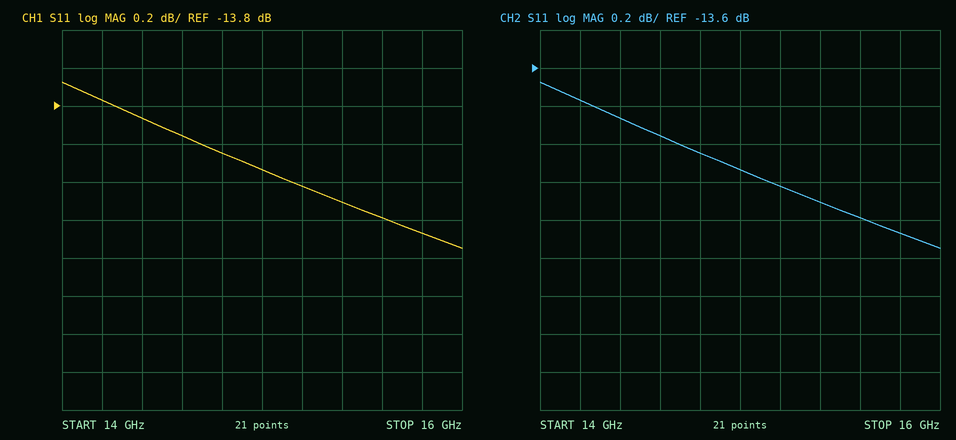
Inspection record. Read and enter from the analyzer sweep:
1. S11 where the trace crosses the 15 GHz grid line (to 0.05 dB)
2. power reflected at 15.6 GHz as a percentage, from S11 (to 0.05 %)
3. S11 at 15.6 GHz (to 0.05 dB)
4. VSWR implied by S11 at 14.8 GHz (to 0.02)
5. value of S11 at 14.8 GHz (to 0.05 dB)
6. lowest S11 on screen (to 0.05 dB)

-14.15 dB
3.65 %
-14.40 dB
1.50
-14.05 dB
-14.55 dB
